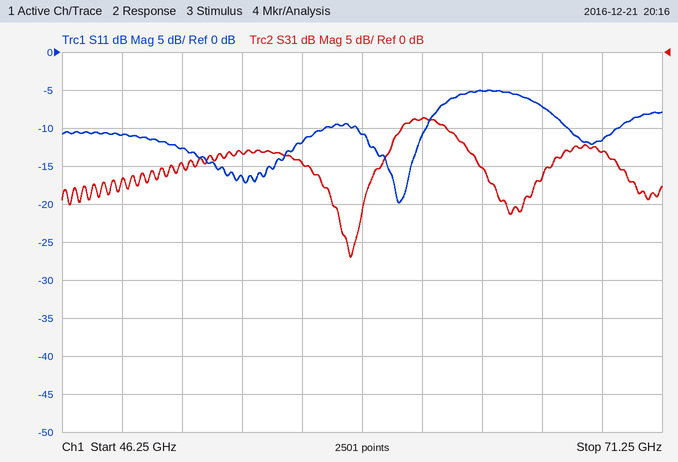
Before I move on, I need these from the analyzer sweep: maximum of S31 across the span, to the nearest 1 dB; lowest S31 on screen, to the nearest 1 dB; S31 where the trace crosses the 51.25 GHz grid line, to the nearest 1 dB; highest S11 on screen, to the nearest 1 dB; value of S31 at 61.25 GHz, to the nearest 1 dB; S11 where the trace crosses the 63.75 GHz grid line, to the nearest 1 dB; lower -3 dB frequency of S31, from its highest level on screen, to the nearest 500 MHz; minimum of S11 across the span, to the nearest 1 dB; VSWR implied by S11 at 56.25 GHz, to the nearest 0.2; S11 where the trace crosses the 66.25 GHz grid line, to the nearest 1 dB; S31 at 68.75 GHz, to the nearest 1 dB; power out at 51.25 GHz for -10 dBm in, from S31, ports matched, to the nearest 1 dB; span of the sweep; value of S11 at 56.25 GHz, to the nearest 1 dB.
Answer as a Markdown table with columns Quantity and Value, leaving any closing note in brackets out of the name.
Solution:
| Quantity | Value |
|---|---|
| maximum of S31 across the span, to the nearest 1 dB | -9 dB |
| lowest S31 on screen, to the nearest 1 dB | -27 dB |
| S31 where the trace crosses the 51.25 GHz grid line, to the nearest 1 dB | -15 dB |
| highest S11 on screen, to the nearest 1 dB | -5 dB |
| value of S31 at 61.25 GHz, to the nearest 1 dB | -9 dB |
| S11 where the trace crosses the 63.75 GHz grid line, to the nearest 1 dB | -5 dB |
| lower -3 dB frequency of S31, from its highest level on screen, to the nearest 500 MHz | 60.0 GHz |
| minimum of S11 across the span, to the nearest 1 dB | -20 dB |
| VSWR implied by S11 at 56.25 GHz, to the nearest 0.2 | 1.6 |
| S11 where the trace crosses the 66.25 GHz grid line, to the nearest 1 dB | -7 dB |
| S31 at 68.75 GHz, to the nearest 1 dB | -13 dB |
| power out at 51.25 GHz for -10 dBm in, from S31, ports matched, to the nearest 1 dB | -25 dBm |
| span of the sweep | 25 GHz |
| value of S11 at 56.25 GHz, to the nearest 1 dB | -12 dB |
